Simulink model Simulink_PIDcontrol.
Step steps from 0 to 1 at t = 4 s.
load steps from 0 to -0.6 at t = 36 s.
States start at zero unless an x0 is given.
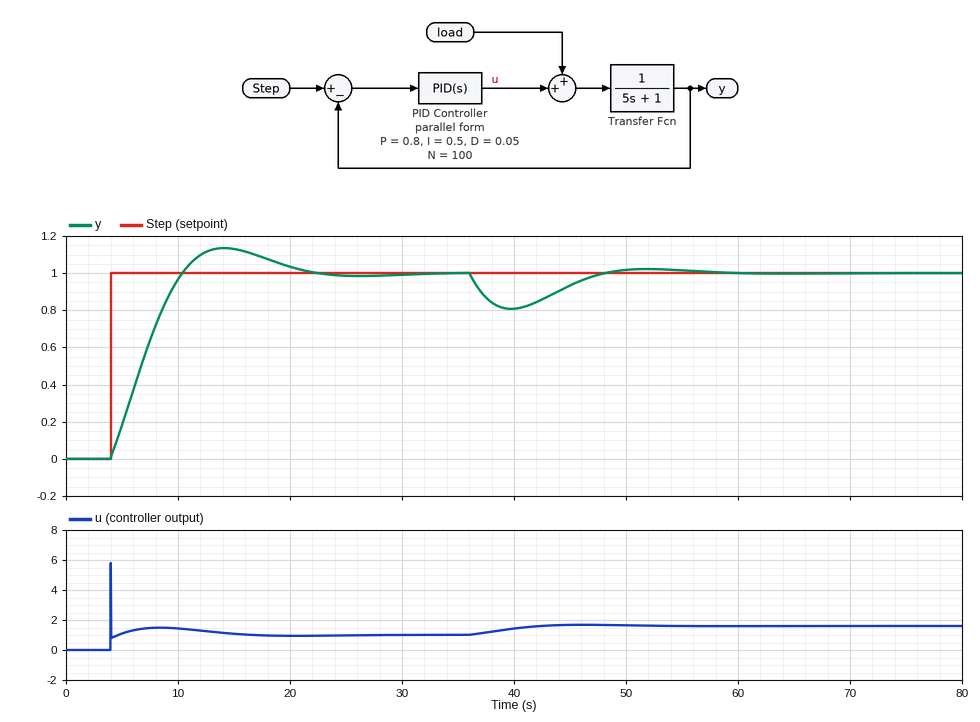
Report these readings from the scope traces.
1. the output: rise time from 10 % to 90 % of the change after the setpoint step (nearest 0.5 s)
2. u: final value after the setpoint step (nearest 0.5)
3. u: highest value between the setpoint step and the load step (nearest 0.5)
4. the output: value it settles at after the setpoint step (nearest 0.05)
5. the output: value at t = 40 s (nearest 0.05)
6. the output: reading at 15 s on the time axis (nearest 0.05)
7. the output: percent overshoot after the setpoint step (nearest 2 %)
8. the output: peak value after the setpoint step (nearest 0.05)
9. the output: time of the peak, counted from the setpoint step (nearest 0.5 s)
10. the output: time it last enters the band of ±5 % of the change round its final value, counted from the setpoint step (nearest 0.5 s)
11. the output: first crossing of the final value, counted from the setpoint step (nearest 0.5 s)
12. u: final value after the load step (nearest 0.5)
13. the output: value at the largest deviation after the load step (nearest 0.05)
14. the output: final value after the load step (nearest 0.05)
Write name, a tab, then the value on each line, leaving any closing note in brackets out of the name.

the output: rise time from 10 % to 90 % of the change after the setpoint step	5.0 s
u: final value after the setpoint step	1.0
u: highest value between the setpoint step and the load step	6.0
the output: value it settles at after the setpoint step	1.00
the output: value at t = 40 s	0.80
the output: reading at 15 s on the time axis	1.15
the output: percent overshoot after the setpoint step	14 %
the output: peak value after the setpoint step	1.15
the output: time of the peak, counted from the setpoint step	10.0 s
the output: time it last enters the band of ±5 % of the change round its final value, counted from the setpoint step	15.0 s
the output: first crossing of the final value, counted from the setpoint step	6.5 s
u: final value after the load step	1.5
the output: value at the largest deviation after the load step	0.80
the output: final value after the load step	1.00
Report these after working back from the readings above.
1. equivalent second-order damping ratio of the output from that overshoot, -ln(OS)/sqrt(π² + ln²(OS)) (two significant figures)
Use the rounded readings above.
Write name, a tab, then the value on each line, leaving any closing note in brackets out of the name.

equivalent second-order damping ratio of the output from that overshoot, -ln(OS)/sqrt(π² + ln²(OS))	0.53
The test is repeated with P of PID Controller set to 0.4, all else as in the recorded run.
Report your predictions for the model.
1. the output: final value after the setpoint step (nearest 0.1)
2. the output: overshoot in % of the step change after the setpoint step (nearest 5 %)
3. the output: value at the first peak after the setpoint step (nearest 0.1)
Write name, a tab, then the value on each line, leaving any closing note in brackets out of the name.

the output: final value after the setpoint step	1.0
the output: overshoot in % of the step change after the setpoint step	20 %
the output: value at the first peak after the setpoint step	1.2
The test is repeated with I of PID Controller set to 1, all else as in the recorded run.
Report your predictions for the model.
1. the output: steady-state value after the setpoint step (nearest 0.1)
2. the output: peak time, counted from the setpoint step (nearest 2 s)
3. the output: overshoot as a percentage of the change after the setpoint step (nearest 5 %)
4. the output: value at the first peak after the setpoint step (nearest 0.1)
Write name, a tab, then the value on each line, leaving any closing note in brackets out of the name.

the output: steady-state value after the setpoint step	1.0
the output: peak time, counted from the setpoint step	6 s
the output: overshoot as a percentage of the change after the setpoint step	25 %
the output: value at the first peak after the setpoint step	1.3
